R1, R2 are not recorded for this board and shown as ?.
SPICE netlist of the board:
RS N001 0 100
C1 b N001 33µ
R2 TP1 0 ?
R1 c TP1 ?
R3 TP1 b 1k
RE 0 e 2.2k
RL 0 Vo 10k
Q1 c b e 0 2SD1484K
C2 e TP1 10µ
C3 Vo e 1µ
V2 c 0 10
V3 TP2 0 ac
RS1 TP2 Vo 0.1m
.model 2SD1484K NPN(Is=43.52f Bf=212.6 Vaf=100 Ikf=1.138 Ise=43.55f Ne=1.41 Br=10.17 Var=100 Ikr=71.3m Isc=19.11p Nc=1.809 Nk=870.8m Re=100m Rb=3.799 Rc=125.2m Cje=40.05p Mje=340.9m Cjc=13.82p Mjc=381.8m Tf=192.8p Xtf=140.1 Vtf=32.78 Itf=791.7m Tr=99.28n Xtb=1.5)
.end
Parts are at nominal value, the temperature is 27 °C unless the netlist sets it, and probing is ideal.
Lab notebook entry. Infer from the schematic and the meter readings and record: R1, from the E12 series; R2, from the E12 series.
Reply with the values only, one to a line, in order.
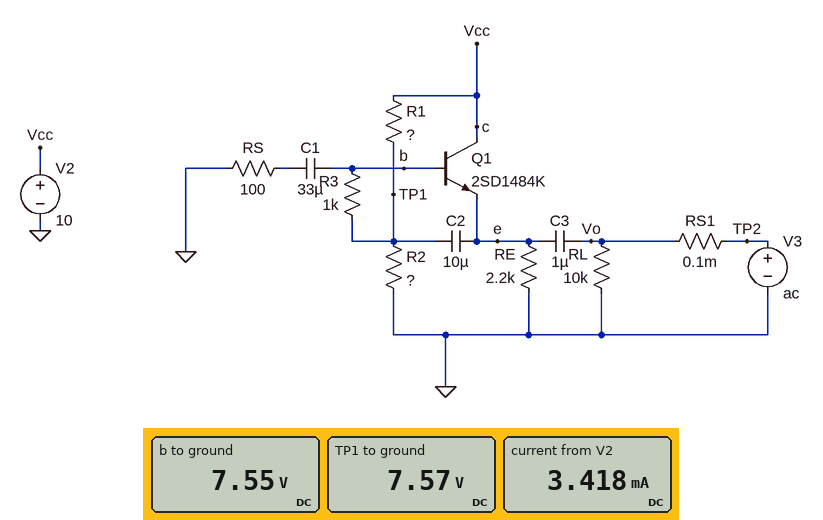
8.2 kΩ
27 kΩ
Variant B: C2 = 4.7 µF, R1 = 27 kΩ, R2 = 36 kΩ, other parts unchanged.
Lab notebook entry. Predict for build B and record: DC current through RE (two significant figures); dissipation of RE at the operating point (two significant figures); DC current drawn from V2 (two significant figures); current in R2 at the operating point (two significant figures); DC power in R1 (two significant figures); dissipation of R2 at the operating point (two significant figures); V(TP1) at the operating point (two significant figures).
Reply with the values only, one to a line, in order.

2.2 mA
11 mW
2.4 mA
150 µA
740 µW
850 µW
5.5 V
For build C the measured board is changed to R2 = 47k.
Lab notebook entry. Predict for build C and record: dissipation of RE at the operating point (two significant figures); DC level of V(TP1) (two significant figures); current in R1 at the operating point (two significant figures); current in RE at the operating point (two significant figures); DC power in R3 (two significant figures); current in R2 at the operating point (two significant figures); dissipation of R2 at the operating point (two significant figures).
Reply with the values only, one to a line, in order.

27 mW
8.4 V
200 µA
3.5 mA
350 nW
180 µA
1.5 mW
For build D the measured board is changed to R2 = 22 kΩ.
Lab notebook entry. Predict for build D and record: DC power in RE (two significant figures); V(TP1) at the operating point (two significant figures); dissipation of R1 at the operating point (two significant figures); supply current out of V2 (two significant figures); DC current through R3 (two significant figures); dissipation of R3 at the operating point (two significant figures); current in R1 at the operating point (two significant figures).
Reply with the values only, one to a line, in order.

19 mW
7.2 V
960 µW
3.3 mA
16 µA
250 nW
340 µA
